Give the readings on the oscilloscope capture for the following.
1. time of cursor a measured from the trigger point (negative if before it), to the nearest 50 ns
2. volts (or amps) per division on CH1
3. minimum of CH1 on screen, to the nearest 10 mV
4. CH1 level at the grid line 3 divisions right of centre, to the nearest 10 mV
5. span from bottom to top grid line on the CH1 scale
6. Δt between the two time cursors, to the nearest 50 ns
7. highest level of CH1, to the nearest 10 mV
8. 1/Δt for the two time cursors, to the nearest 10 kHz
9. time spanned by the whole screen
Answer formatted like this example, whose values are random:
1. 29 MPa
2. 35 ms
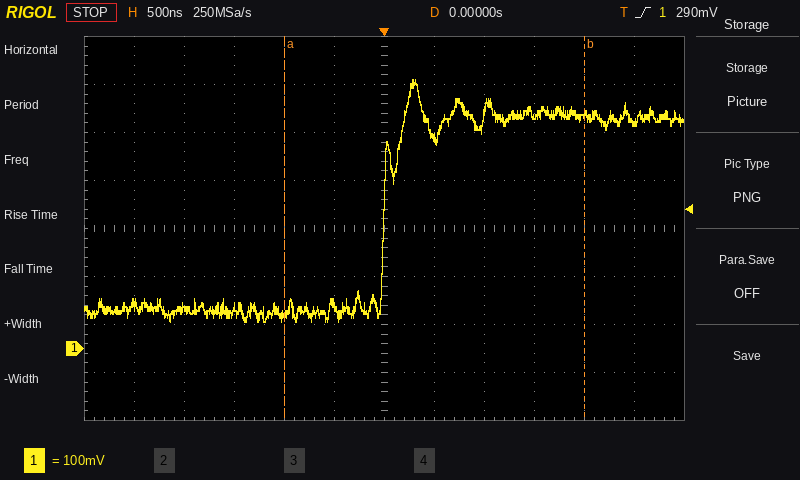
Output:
1. -1.00 µs
2. 100 mV
3. 60 mV
4. 490 mV
5. 800 mV
6. 3.00 µs
7. 560 mV
8. 330 kHz
9. 6 µs
